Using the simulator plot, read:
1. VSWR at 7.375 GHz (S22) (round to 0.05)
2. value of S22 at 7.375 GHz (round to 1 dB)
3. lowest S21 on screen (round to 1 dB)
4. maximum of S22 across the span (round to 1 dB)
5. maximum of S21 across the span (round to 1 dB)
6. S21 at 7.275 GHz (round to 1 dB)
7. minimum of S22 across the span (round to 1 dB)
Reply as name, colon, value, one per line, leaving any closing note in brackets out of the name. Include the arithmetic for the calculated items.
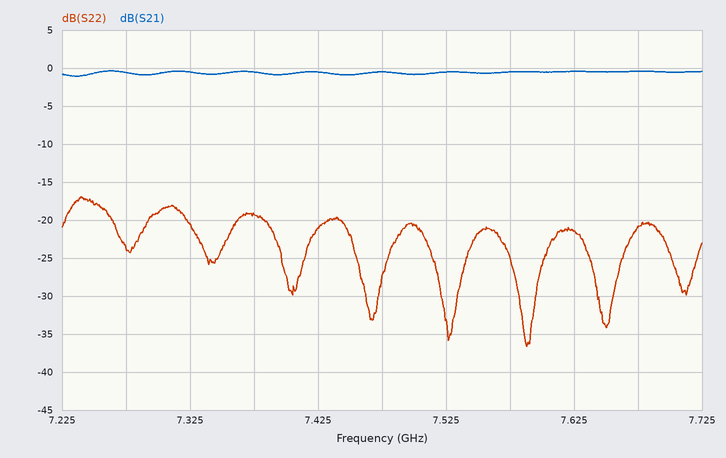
VSWR at 7.375 GHz (S22): |Γ| = 10^(-19/20) = 0.1122; VSWR = (1 + 0.1122)/(1 − 0.1122) ≈ 1.25
value of S22 at 7.375 GHz: -19 dB
lowest S21 on screen: -1 dB
maximum of S22 across the span: -17 dB
maximum of S21 across the span: 0 dB
S21 at 7.275 GHz: -1 dB
minimum of S22 across the span: -37 dB
